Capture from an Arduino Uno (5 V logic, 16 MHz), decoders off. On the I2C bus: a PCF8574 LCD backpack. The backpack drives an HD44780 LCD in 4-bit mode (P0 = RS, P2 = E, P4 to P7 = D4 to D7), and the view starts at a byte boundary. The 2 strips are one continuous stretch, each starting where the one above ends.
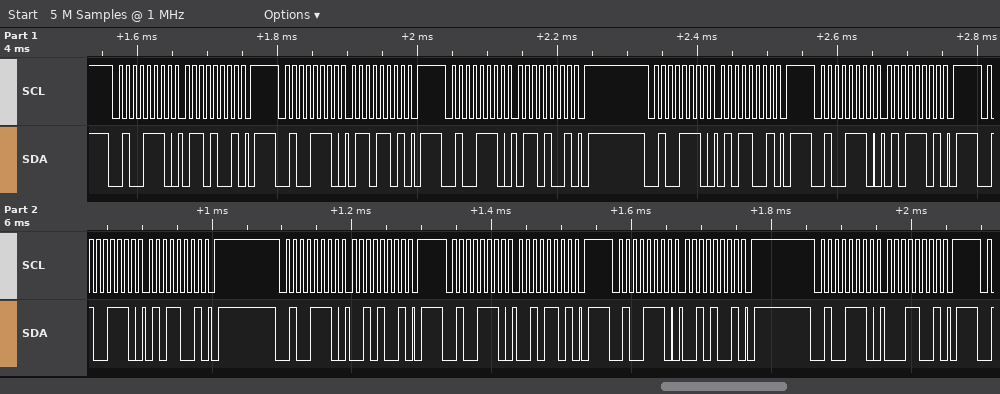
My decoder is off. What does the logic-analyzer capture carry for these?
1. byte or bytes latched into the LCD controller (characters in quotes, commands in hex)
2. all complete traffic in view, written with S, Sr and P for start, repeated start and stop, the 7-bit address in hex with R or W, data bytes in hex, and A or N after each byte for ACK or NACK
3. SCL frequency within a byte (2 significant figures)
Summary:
'e'
S 27W A 69 A P S 27W A 6D A P S 27W A 69 A P S 27W A 59 A P S 27W A 5D A P S 27W A 59 A P S 27W A 29 A P S 27W A 2D A P S 27W A 29 A P S 27W A 19 A P
100 kHz
